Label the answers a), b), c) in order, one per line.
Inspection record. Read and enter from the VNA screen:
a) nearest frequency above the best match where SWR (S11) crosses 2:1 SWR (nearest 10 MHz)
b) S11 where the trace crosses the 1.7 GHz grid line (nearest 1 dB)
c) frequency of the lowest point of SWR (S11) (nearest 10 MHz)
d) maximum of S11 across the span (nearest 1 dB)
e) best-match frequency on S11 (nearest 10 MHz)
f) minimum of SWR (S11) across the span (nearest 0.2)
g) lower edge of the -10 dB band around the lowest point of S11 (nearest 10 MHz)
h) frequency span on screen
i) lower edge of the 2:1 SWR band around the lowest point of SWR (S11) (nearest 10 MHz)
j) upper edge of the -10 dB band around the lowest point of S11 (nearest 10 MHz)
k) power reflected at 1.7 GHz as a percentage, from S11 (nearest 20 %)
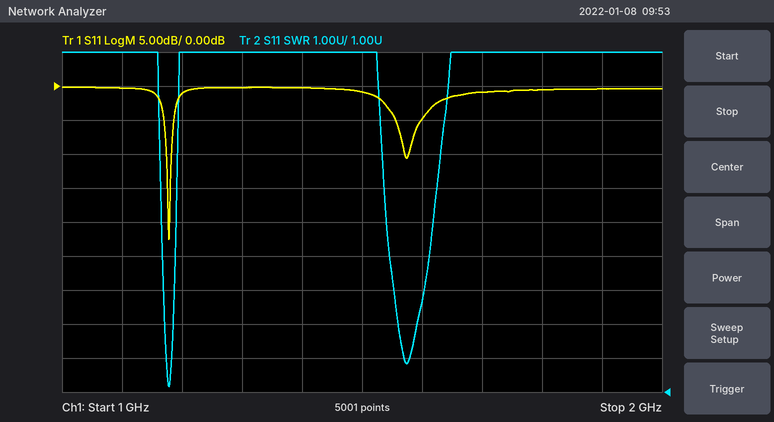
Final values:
a) 1.18 GHz
b) -1 dB
c) 1.18 GHz
d) 0 dB
e) 1.18 GHz
f) 1.2
g) 1.17 GHz
h) 1 GHz
i) 1.17 GHz
j) 1.18 GHz
k) 80 %
